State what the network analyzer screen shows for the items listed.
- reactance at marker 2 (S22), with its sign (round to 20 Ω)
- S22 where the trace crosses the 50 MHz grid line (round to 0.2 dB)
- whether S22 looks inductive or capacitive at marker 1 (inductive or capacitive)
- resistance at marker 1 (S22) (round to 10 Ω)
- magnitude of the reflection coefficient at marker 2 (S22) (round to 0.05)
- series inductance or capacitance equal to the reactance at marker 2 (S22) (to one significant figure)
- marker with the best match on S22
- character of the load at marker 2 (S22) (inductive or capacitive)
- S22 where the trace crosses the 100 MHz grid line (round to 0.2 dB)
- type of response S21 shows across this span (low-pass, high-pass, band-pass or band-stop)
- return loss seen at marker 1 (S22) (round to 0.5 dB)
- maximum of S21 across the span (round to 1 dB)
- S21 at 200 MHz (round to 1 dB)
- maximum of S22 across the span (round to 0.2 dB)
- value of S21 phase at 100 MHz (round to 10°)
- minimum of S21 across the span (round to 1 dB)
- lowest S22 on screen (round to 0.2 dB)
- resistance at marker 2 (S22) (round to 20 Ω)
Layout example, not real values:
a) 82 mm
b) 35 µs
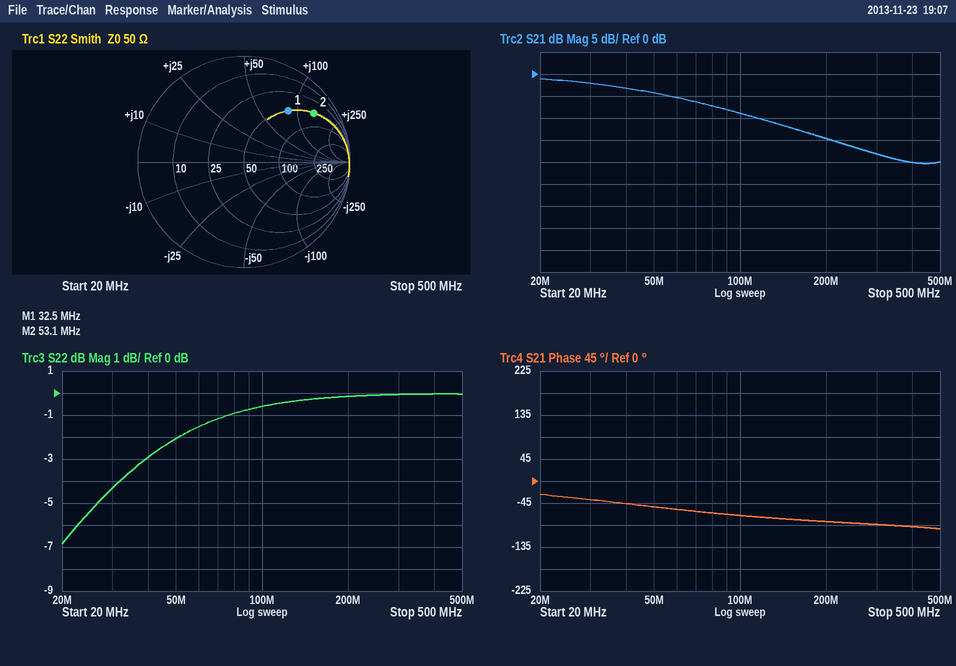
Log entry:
a) +140 Ω
b) -2.0 dB
c) inductive
d) 50 Ω
e) 0.80
f) 400 nH
g) marker 1
h) inductive
i) -0.6 dB
j) low-pass
k) 4.0 dB
l) -1 dB
m) -15 dB
n) 0.0 dB
o) -70°
p) -20 dB
q) -6.8 dB
r) 60 Ω
